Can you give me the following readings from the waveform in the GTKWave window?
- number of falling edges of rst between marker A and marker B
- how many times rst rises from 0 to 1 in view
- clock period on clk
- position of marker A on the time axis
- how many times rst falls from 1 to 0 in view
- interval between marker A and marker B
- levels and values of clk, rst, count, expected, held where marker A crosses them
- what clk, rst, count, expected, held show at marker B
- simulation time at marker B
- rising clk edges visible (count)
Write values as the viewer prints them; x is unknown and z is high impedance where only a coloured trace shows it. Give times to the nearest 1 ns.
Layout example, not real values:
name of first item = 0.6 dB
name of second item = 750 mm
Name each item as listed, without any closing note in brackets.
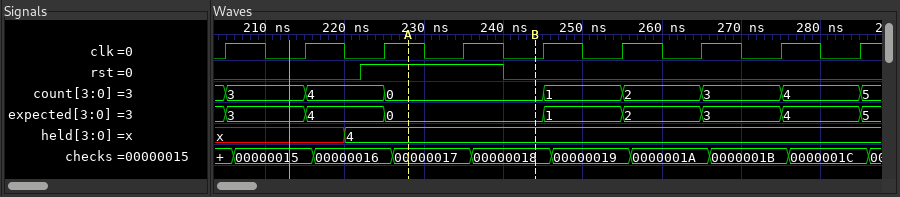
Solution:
number of falling edges of rst between marker A and marker B = 1
how many times rst rises from 0 to 1 in view = 1
clock period on clk = 10 ns
position of marker A on the time axis = 228 ns
how many times rst falls from 1 to 0 in view = 1
interval between marker A and marker B = 16 ns
levels and values of clk, rst, count, expected, held where marker A crosses them = clk=1, rst=1, count=0, expected=0, held=4
what clk, rst, count, expected, held show at marker B = clk=0, rst=0, count=0, expected=0, held=4
simulation time at marker B = 244 ns
rising clk edges visible = 9
